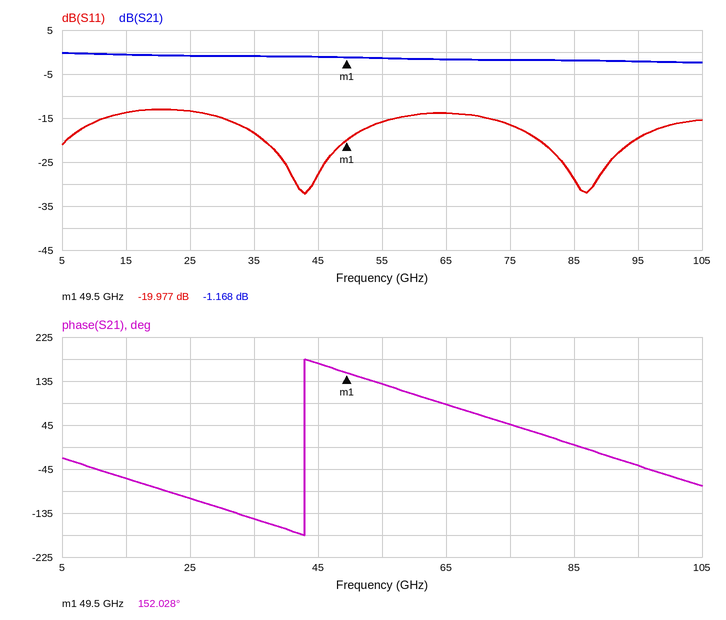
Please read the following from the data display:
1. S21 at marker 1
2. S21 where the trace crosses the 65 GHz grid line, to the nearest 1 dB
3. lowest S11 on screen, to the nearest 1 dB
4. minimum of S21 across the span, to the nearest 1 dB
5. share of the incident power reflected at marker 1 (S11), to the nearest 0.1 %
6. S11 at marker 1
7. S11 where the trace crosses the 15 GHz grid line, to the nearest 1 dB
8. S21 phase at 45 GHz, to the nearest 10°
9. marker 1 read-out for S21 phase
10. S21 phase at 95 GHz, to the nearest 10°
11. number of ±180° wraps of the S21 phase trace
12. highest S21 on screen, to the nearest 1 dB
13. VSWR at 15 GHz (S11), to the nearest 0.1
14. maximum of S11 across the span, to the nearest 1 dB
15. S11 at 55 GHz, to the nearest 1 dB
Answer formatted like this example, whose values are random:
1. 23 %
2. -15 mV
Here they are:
1. -1.168 dB
2. -2 dB
3. -32 dB
4. -2 dB
5. 1.0 %
6. -19.977 dB
7. -14 dB
8. 170°
9. 152.028°
10. -40°
11. 1
12. 0 dB
13. 1.5
14. -13 dB
15. -16 dB
